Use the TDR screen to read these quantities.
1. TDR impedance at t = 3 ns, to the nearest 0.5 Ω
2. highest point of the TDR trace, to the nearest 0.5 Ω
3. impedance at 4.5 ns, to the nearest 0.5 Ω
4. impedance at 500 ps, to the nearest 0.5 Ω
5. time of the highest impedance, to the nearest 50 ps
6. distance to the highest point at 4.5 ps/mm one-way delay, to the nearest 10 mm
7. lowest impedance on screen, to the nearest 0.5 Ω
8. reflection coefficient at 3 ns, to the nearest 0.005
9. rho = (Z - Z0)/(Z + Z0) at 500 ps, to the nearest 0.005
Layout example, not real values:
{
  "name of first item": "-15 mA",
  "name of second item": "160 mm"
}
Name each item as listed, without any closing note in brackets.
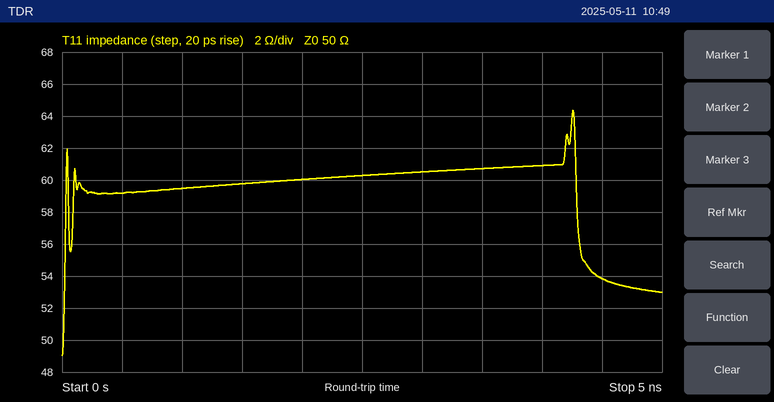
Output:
{
  "TDR impedance at t = 3 ns, to the nearest 0.5 Ω": "60.5 Ω",
  "highest point of the TDR trace, to the nearest 0.5 Ω": "64.5 Ω",
  "impedance at 4.5 ns, to the nearest 0.5 Ω": "54.0 Ω",
  "impedance at 500 ps, to the nearest 0.5 Ω": "59.0 Ω",
  "time of the highest impedance, to the nearest 50 ps": "4.25 ns",
  "distance to the highest point at 4.5 ps/mm one-way delay, to the nearest 10 mm": "470 mm",
  "lowest impedance on screen, to the nearest 0.5 Ω": "49.0 Ω",
  "reflection coefficient at 3 ns, to the nearest 0.005": "+0.095",
  "rho = (Z - Z0)/(Z + Z0) at 500 ps, to the nearest 0.005": "+0.085"
}
